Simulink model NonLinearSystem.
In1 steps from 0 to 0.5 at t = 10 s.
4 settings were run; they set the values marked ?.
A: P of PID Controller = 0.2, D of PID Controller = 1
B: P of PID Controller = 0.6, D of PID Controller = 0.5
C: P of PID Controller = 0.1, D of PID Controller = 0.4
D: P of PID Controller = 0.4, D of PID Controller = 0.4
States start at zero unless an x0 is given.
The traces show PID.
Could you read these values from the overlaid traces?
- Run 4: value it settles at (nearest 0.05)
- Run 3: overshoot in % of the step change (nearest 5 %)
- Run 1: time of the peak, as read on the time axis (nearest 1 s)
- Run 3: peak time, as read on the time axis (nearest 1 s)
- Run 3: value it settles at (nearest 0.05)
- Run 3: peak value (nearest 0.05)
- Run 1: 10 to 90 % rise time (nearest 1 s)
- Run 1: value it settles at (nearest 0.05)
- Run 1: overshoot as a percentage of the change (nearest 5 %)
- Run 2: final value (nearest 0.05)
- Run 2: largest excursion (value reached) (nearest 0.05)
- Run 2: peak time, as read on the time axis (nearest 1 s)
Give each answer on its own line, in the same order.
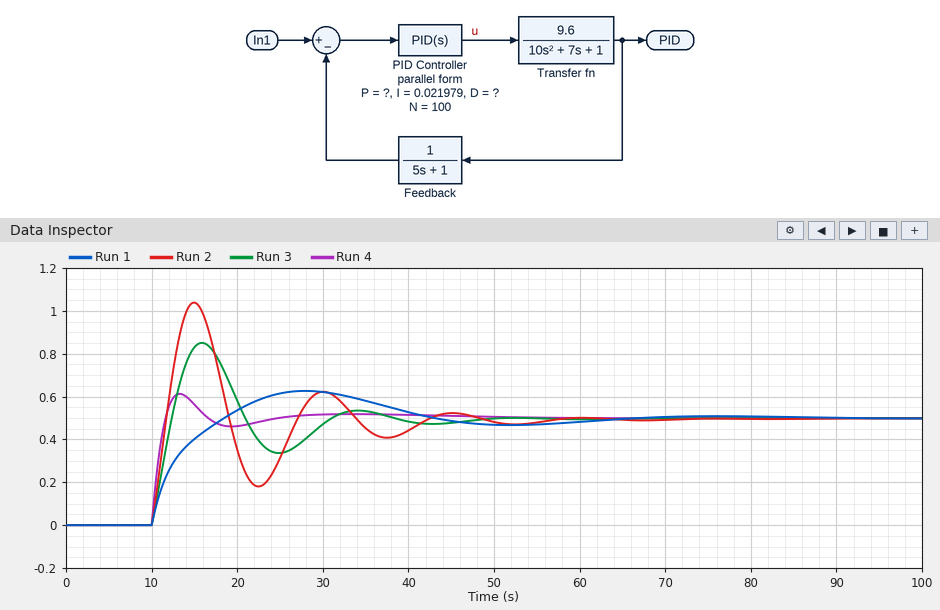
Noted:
0.50
70 %
28 s
16 s
0.50
0.85
6 s
0.50
25 %
0.50
1.05
15 s
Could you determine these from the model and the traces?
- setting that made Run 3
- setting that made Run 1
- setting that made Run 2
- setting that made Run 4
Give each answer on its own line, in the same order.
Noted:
D
C
B
A
